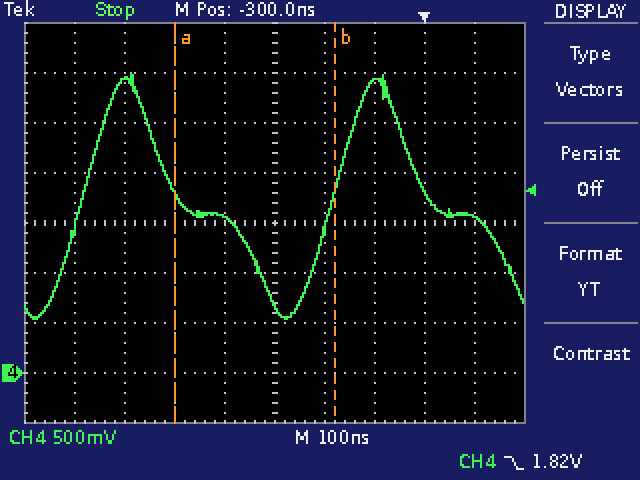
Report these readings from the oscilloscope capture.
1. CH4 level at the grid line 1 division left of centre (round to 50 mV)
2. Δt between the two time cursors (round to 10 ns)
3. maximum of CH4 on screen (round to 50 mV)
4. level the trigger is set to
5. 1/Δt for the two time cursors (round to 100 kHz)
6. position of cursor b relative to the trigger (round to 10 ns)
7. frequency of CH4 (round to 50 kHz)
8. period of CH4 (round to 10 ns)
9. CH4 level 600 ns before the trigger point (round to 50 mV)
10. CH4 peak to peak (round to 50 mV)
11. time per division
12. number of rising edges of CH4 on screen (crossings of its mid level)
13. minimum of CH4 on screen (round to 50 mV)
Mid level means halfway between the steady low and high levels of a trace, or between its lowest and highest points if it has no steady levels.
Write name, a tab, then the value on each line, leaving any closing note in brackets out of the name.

CH4 level at the grid line 1 division left of centre	1.55 V
Δt between the two time cursors	320 ns
maximum of CH4 on screen	3.00 V
level the trigger is set to	1.82 V
1/Δt for the two time cursors	3.1 MHz
position of cursor b relative to the trigger	-180 ns
frequency of CH4	2.00 MHz
period of CH4	500 ns
CH4 level 600 ns before the trigger point	2.95 V
CH4 peak to peak	2.45 V
time per division	100 ns
number of rising edges of CH4 on screen	2
minimum of CH4 on screen	550 mV
